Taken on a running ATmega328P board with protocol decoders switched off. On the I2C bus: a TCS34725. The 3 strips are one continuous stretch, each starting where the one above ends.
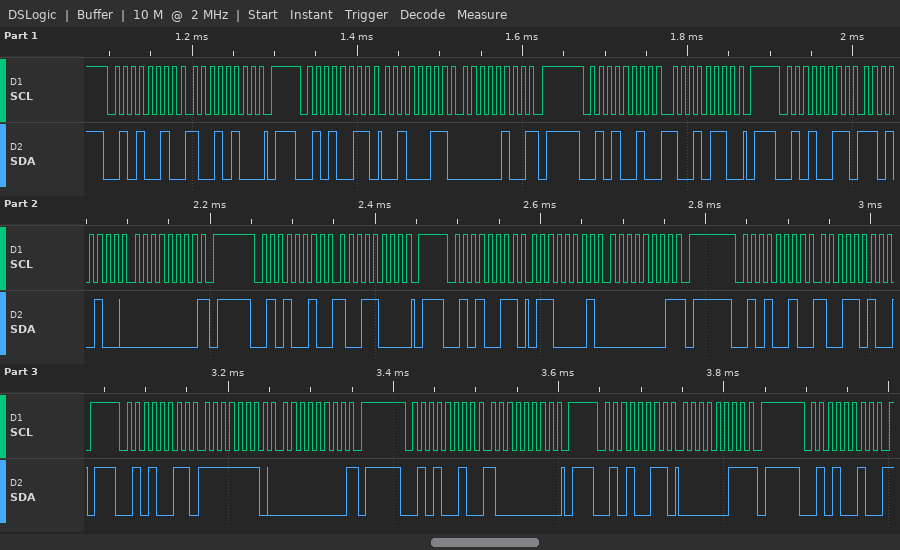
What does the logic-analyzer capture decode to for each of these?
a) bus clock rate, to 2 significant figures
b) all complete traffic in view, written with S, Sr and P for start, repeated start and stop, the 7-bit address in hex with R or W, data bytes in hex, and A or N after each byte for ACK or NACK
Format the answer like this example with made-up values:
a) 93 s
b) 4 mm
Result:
a) 100 kHz
b) S 29W A 94 A P S 29R A 23 A 04 N P S 29W A 96 A P S 29R A D4 A 00 N P S 29W A 98 A P S 29R A 61 A 01 N P S 29W A 9A A P S 29R A FE A 00 N P S 29W A 80 A P S 29R A 03 N P S 29W A
